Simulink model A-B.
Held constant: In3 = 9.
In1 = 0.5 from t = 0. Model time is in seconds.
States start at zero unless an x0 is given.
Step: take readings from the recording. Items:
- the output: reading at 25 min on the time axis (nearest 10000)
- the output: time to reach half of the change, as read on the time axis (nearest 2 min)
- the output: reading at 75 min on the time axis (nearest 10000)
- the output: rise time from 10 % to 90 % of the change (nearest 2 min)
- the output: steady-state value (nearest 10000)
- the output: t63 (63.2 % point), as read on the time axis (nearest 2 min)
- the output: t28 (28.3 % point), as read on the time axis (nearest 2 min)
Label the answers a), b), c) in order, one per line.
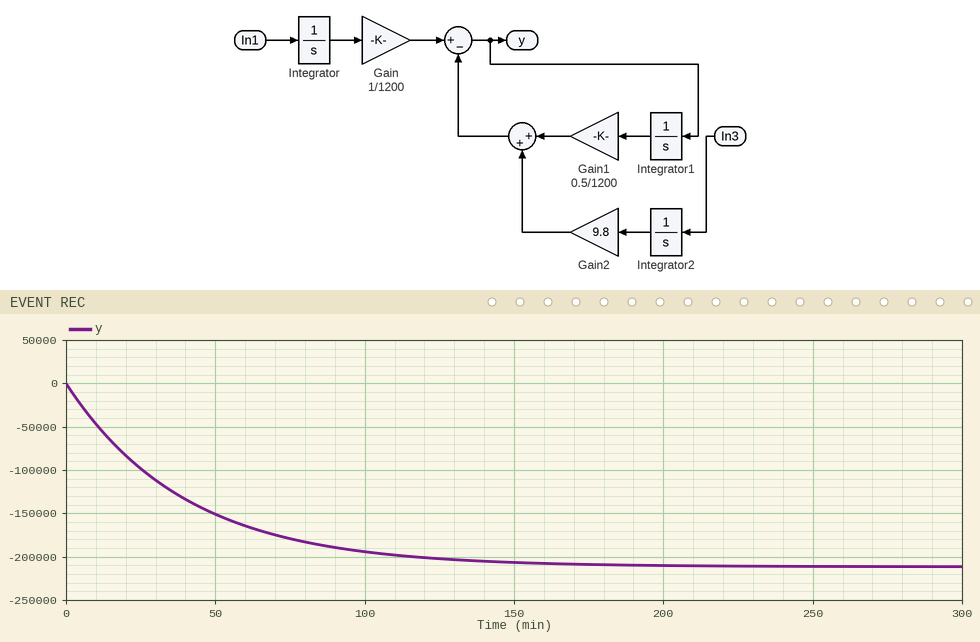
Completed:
a) -100000
b) 28 min
c) -180000
d) 88 min
e) -210000
f) 40 min
g) 14 min
